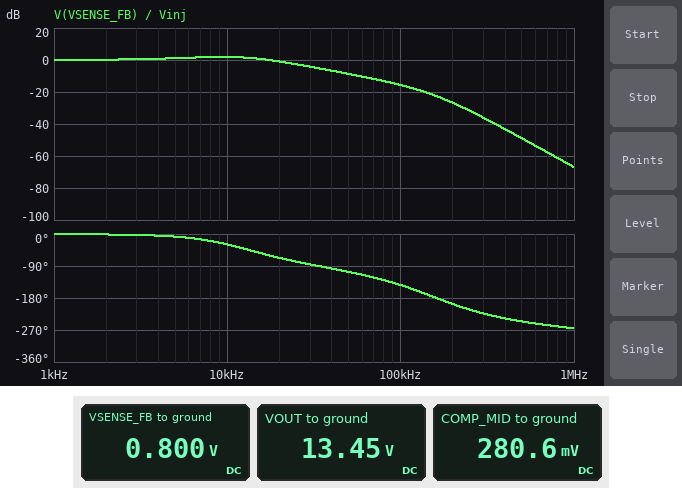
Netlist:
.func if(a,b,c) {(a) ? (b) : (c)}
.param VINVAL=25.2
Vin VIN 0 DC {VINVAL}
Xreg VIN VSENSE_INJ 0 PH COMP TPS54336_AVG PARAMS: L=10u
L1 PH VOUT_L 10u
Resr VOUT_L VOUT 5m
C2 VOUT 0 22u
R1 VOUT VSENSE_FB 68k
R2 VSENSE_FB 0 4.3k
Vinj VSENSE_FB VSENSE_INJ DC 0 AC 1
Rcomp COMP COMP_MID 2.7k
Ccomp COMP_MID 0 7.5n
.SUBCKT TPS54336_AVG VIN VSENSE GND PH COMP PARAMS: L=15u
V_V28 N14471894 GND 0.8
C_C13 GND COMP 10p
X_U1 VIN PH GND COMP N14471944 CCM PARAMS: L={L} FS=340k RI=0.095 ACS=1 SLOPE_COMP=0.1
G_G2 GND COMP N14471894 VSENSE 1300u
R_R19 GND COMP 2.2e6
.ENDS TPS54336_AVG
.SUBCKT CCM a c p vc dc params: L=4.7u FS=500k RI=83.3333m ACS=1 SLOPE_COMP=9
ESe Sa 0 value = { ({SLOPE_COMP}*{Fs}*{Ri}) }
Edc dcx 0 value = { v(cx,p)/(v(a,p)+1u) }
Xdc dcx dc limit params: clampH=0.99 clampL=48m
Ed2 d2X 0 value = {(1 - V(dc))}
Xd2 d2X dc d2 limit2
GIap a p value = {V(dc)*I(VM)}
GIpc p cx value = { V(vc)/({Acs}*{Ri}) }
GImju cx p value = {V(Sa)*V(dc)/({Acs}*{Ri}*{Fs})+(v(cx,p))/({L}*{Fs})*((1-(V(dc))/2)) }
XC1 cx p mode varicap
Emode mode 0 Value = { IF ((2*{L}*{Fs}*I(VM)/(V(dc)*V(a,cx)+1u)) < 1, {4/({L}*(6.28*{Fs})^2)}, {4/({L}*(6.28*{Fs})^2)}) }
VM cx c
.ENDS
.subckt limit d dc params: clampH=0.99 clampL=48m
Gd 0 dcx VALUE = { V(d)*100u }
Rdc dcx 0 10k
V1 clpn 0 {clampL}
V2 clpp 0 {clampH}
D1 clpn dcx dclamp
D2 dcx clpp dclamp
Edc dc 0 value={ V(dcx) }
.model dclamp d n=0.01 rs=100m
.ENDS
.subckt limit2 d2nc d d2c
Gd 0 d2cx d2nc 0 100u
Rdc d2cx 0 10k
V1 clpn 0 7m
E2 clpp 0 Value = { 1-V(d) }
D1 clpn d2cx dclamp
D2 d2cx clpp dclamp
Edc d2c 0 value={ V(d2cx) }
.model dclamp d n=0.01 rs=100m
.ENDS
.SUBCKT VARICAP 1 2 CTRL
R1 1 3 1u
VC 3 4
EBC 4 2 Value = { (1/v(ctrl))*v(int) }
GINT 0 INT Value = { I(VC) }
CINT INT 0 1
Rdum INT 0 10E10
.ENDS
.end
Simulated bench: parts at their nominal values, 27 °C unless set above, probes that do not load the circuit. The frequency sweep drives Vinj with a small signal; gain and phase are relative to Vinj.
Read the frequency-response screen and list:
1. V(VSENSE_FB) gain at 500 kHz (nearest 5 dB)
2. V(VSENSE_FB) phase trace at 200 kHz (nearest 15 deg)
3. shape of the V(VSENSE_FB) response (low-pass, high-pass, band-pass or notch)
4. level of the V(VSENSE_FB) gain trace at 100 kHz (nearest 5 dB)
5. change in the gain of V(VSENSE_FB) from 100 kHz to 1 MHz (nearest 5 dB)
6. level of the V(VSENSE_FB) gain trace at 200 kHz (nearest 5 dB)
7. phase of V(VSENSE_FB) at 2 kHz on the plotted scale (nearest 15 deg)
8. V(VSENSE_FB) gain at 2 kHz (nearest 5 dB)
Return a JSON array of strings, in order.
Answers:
["-50 dB", "-195 deg", "low-pass", "-15 dB", "-50 dB", "-25 dB", "0 deg", "0 dB"]
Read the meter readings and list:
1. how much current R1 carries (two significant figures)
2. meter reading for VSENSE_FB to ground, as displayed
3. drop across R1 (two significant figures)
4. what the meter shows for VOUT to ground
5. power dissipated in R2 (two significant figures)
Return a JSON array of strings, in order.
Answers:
["190 µA", "0.800 V", "13 V", "13.45 V", "150 µW"]
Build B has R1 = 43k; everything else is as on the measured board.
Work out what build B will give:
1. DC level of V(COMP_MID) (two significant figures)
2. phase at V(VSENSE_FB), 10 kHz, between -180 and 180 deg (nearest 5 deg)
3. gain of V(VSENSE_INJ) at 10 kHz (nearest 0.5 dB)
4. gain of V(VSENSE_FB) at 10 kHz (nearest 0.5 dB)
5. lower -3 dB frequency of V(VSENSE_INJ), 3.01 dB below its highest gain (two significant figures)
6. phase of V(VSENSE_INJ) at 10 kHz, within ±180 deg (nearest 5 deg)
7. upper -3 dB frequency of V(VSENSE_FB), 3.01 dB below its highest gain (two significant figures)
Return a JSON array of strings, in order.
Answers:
["210 mV", "-20 deg", "-8.5 dB", "1.5 dB", "21 kHz", "-70 deg", "34 kHz"]
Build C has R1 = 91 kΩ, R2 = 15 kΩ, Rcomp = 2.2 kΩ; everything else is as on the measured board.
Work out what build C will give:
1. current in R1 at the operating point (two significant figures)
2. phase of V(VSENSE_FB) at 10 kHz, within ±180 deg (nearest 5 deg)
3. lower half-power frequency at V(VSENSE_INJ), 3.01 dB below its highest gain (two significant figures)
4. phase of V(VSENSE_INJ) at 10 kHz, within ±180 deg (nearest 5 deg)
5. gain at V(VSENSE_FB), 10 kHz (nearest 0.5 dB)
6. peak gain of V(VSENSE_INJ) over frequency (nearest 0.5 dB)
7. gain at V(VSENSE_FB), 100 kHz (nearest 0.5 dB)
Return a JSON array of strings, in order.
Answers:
["53 µA", "-10 deg", "26 kHz", "-60 deg", "1.5 dB", "3.0 dB", "-12.5 dB"]
